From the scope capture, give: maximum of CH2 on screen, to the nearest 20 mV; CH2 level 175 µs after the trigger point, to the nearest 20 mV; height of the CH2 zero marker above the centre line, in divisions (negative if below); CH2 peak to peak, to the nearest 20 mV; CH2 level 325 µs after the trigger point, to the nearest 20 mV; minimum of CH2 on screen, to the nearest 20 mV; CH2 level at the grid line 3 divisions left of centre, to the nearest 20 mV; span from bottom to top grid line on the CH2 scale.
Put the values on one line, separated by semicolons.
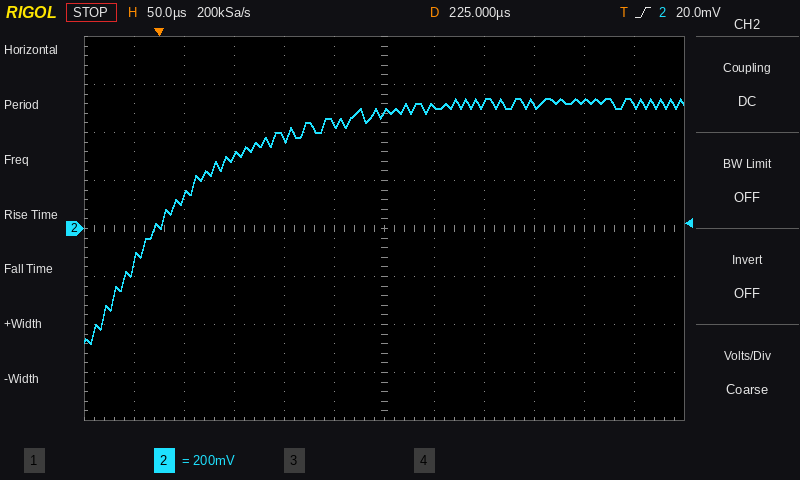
540 mV; 440 mV; 0.0 div; 1.02 V; 520 mV; -480 mV; 300 mV; 1.6 V
